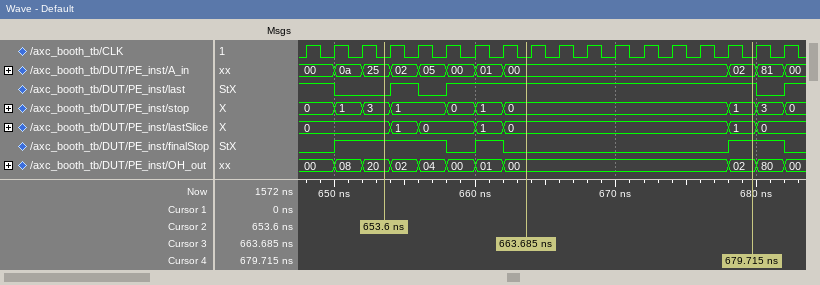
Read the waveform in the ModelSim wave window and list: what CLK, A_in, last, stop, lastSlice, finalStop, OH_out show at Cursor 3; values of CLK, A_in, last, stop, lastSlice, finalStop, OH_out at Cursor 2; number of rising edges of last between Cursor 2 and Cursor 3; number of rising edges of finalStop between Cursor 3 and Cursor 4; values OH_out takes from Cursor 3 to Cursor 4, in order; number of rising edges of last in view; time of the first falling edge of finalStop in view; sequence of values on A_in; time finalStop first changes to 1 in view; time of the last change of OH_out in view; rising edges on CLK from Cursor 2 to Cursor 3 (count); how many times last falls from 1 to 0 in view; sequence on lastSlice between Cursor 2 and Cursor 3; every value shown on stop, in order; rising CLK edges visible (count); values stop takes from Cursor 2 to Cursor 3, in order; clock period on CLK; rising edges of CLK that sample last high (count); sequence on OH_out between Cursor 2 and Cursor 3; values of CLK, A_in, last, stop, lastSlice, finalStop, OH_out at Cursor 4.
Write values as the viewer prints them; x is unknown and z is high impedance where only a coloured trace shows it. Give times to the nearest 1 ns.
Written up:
CLK=0, A_in=00, last=1, stop=0, lastSlice=0, finalStop=0, OH_out=00
CLK=0, A_in=25, last=0, stop=3, lastSlice=0, finalStop=1, OH_out=20
2
1
00, 02
3
658 ns
00, 0a, 25, 02, 05, 00, 01, 00, 02, 81, 00
650 ns
682 ns
5
3
0, 1, 0, 1, 0
0, 1, 3, 1, 0, 1, 0, 1, 3, 0
18
3, 1, 0, 1, 0
2 ns
14
20, 02, 04, 00, 01, 00
CLK=0, A_in=02, last=1, stop=1, lastSlice=1, finalStop=1, OH_out=02
